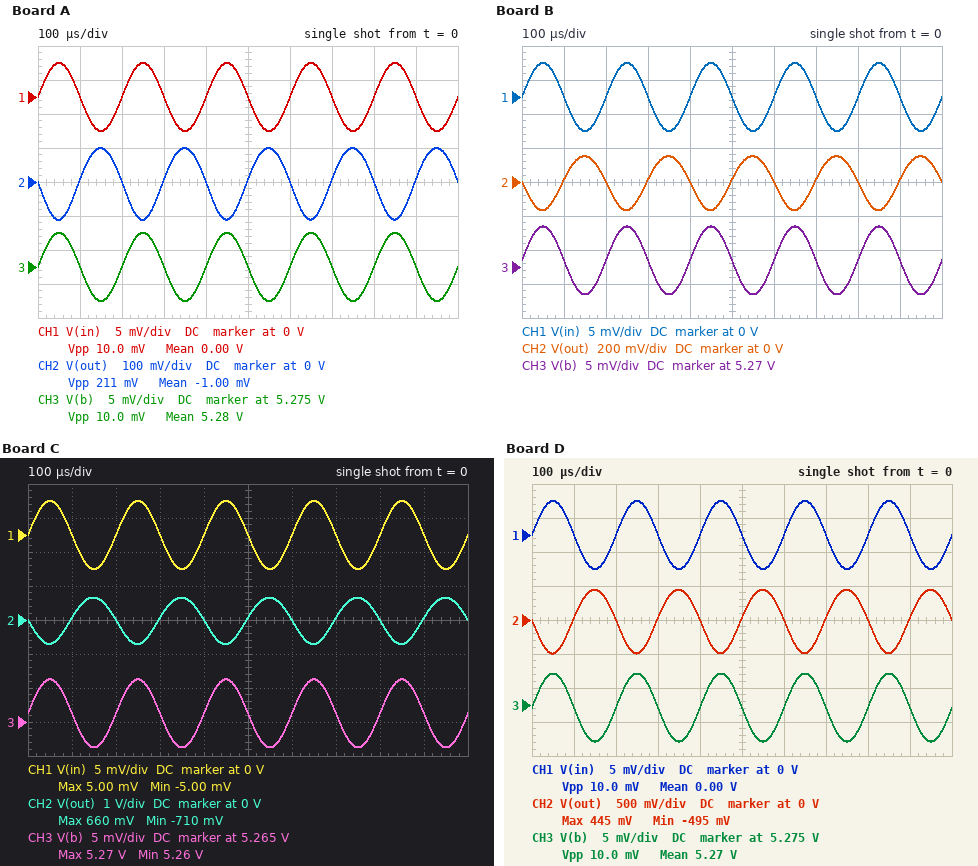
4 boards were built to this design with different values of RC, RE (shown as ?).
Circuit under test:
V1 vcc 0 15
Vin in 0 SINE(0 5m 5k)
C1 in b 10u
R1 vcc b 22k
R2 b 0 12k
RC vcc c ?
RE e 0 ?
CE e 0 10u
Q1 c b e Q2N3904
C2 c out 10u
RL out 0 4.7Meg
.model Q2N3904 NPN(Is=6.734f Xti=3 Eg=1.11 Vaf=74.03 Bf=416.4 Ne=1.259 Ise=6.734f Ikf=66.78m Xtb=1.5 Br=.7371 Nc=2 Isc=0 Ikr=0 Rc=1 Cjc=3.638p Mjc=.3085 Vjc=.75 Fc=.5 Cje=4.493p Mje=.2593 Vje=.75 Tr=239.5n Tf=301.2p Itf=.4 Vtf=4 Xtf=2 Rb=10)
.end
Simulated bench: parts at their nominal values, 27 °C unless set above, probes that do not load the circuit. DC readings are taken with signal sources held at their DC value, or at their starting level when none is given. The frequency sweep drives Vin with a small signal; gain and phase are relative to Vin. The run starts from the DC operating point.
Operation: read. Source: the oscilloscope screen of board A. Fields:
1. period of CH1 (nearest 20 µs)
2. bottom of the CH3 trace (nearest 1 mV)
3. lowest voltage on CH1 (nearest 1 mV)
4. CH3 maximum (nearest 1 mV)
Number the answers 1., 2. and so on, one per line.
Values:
1. 200 µs
2. 5.270 V
3. -5 mV
4. 5.280 V
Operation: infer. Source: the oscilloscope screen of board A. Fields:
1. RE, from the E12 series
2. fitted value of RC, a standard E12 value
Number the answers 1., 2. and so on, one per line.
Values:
1. 15 kΩ
2. 1.8 kΩ
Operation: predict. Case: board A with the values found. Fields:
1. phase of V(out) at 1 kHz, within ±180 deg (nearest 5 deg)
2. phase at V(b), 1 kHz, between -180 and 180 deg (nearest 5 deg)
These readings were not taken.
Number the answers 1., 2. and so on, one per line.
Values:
1. -170 deg
2. 0 deg
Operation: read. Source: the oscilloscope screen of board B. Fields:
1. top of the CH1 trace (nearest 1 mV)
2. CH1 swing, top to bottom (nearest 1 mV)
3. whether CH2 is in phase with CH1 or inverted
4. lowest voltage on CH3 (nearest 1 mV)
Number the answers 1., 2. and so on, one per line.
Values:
1. 5 mV
2. 10 mV
3. inverted
4. 5.266 V
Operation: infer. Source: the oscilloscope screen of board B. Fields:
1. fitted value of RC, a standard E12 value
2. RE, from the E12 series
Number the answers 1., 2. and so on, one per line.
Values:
1. 2.2 kΩ
2. 12 kΩ
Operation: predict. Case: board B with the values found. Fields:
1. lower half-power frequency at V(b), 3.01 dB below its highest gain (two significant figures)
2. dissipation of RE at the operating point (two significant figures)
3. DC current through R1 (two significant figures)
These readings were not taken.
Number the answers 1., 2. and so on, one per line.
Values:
1. 2.1 Hz
2. 1.8 mW
3. 440 µA
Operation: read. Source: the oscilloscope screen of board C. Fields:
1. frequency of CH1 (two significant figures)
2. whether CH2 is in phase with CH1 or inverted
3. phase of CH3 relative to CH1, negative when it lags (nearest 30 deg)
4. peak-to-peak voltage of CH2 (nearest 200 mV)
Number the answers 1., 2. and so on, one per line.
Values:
1. 5.0 kHz
2. inverted
3. 0 deg
4. 1.4 V
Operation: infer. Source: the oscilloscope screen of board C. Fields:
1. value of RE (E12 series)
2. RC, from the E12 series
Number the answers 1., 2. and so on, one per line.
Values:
1. 10 kΩ
2. 8.2 kΩ
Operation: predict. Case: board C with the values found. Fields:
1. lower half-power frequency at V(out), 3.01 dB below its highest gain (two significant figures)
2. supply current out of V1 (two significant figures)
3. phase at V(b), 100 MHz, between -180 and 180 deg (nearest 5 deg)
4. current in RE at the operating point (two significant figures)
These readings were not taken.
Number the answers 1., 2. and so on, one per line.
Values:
1. 270 Hz
2. 900 µA
3. 0 deg
4. 460 µA
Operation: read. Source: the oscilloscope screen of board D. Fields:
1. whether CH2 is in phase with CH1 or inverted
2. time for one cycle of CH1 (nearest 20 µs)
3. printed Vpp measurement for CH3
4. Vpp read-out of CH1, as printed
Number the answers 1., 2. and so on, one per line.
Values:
1. inverted
2. 200 µs
3. 10.0 mV
4. 10.0 mV
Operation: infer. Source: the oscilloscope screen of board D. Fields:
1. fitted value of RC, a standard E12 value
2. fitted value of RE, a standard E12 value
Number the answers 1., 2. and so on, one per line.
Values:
1. 8.2 kΩ
2. 15 kΩ
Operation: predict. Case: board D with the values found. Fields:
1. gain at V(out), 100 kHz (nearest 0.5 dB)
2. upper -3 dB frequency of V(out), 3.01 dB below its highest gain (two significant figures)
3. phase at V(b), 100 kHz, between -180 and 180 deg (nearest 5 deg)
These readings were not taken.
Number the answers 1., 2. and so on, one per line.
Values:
1. 39.5 dB
2. 10 MHz
3. 0 deg
